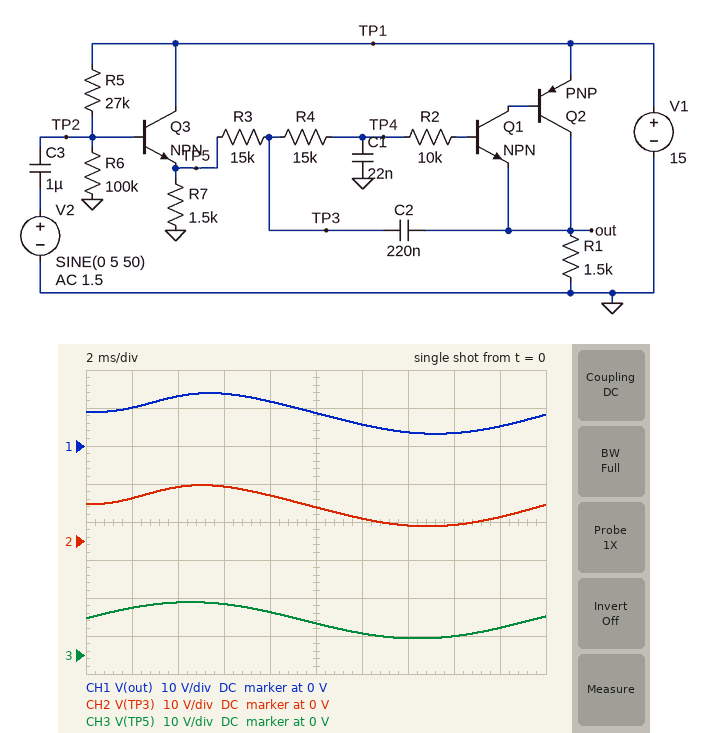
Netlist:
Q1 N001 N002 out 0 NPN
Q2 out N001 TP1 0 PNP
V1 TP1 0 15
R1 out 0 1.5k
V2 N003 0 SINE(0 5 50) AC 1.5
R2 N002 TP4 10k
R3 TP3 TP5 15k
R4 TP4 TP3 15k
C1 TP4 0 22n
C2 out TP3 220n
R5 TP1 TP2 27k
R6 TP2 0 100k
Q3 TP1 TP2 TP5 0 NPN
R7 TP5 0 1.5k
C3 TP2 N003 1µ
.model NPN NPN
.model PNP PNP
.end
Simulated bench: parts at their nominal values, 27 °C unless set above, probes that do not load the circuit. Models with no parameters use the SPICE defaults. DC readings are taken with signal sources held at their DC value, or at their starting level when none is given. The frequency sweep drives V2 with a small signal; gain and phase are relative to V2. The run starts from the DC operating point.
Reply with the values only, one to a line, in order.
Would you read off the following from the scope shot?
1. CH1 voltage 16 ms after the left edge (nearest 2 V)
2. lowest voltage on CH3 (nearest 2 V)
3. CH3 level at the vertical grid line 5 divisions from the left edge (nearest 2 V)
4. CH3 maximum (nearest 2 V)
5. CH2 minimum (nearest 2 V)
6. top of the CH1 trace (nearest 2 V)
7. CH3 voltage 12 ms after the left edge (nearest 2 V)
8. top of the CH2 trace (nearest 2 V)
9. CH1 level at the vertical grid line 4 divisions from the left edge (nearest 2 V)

4 V
4 V
8 V
14 V
4 V
14 V
6 V
14 V
12 V
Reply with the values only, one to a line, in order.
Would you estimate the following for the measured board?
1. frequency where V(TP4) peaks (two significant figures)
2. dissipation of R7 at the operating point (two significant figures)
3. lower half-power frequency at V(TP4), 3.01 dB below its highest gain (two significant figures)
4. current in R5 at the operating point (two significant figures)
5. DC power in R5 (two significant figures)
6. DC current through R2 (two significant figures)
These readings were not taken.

140 Hz
62 mW
66 Hz
170 µA
760 µW
590 nA
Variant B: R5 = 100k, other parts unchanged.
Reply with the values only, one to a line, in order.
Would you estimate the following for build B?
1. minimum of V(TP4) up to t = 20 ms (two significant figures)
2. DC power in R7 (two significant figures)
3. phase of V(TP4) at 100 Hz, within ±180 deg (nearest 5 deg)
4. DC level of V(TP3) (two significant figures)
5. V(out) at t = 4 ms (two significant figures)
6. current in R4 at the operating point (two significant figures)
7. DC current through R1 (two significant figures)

190 mV
17 mW
-35 deg
5.0 V
8.6 V
290 nA
2.9 mA
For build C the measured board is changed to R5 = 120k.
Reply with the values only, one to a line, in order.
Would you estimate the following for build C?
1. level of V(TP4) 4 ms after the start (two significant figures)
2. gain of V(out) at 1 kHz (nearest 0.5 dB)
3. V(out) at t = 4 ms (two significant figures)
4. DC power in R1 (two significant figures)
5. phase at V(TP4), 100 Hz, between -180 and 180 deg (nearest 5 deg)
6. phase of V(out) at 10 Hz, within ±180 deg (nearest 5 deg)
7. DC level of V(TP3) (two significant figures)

8.7 V
-33.0 dB
8.0 V
9.3 mW
-35 deg
20 deg
4.4 V
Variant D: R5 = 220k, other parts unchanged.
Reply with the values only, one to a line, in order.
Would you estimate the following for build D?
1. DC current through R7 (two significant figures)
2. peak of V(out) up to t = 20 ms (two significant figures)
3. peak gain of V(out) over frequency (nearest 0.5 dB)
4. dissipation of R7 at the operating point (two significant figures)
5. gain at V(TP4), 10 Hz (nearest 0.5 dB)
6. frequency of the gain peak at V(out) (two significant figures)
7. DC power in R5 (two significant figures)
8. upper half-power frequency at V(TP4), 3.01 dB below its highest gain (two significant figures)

1.8 mA
7.4 V
3.5 dB
4.8 mW
-0.5 dB
130 Hz
600 µW
180 Hz
